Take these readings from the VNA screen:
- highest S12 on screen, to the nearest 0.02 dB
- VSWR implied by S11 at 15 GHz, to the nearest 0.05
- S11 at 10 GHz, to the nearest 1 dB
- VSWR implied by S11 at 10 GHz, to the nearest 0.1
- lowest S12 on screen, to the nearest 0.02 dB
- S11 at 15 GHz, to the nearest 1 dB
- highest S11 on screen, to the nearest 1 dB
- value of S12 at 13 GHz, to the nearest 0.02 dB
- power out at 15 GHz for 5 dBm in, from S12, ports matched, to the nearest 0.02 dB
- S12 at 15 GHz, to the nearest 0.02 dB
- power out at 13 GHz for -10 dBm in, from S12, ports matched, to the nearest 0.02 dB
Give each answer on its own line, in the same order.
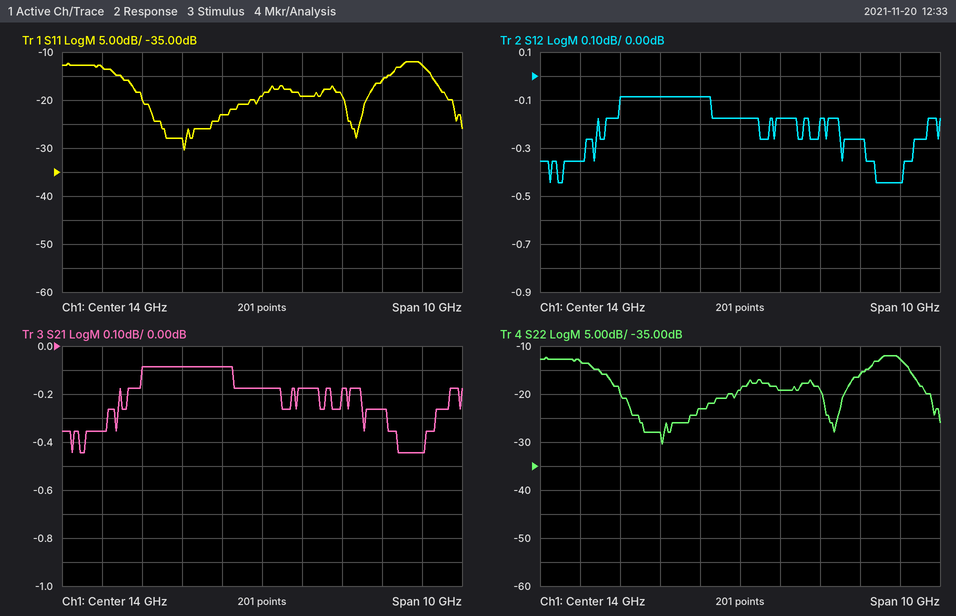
-0.08 dB
1.25
-13 dB
1.6
-0.44 dB
-19 dB
-12 dB
-0.08 dB
4.82 dBm
-0.18 dB
-10.08 dBm
